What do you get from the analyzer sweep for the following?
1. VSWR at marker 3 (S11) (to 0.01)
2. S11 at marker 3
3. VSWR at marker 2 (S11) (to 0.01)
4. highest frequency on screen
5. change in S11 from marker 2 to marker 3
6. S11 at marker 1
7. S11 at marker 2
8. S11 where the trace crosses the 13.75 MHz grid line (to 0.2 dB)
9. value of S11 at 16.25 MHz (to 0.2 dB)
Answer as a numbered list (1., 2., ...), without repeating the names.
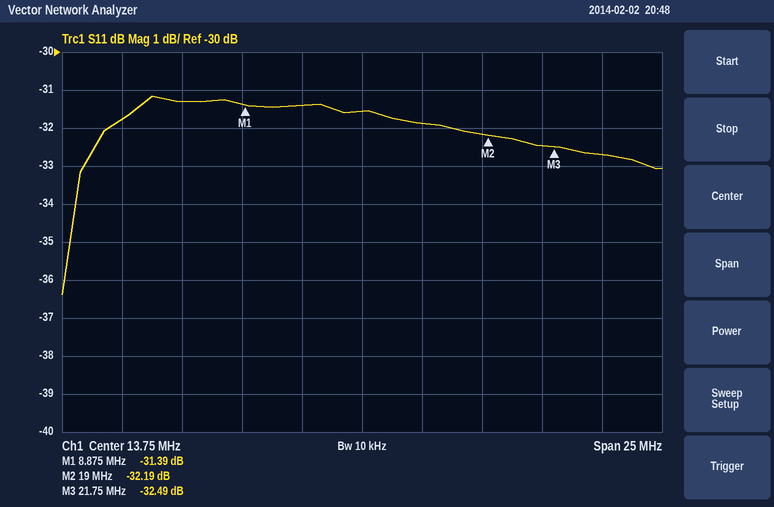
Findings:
1. 1.05
2. -32.49 dB
3. 1.05
4. 26.25 MHz
5. -0.30 dB
6. -31.39 dB
7. -32.19 dB
8. -31.6 dB
9. -31.8 dB
